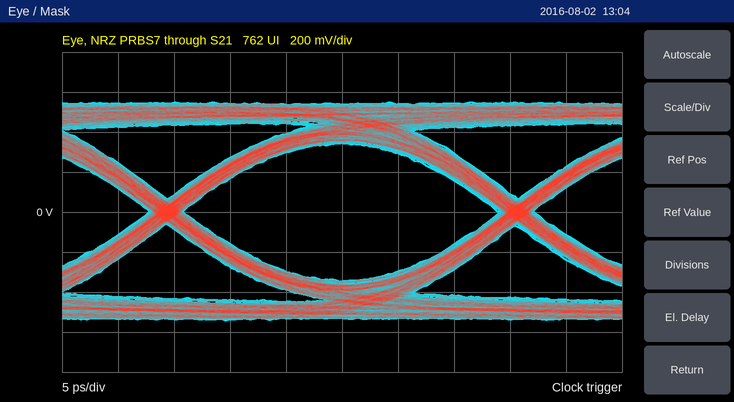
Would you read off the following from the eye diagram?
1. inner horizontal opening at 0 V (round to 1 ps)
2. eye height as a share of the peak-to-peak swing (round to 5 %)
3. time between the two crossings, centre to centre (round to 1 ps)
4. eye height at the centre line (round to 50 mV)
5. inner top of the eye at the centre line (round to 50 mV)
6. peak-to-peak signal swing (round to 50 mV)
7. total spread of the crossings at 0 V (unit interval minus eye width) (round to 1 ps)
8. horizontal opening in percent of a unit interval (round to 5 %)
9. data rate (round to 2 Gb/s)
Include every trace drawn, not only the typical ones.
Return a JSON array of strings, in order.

["28 ps", "65 %", "31 ps", "700 mV", "350 mV", "1.10 V", "3 ps", "90 %", "32 Gb/s"]
